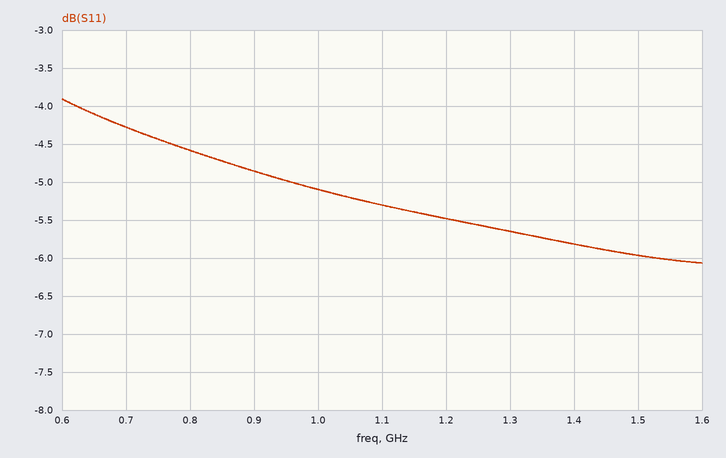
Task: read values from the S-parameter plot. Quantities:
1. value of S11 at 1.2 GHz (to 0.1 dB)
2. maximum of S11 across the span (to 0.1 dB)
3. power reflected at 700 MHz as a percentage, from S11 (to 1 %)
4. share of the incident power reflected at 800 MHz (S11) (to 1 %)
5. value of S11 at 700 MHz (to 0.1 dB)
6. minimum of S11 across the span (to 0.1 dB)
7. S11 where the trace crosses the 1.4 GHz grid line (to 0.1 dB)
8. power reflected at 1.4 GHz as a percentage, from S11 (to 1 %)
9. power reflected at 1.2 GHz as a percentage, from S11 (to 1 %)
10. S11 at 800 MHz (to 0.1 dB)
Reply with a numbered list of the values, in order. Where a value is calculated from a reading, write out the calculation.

1. -5.5 dB
2. -3.9 dB
3. 10^(-4.3/10) ≈ 37 %
4. 10^(-4.6/10) ≈ 35 %
5. -4.3 dB
6. -6.1 dB
7. -5.8 dB
8. 10^(-5.8/10) ≈ 26 %
9. 10^(-5.5/10) ≈ 28 %
10. -4.6 dB
